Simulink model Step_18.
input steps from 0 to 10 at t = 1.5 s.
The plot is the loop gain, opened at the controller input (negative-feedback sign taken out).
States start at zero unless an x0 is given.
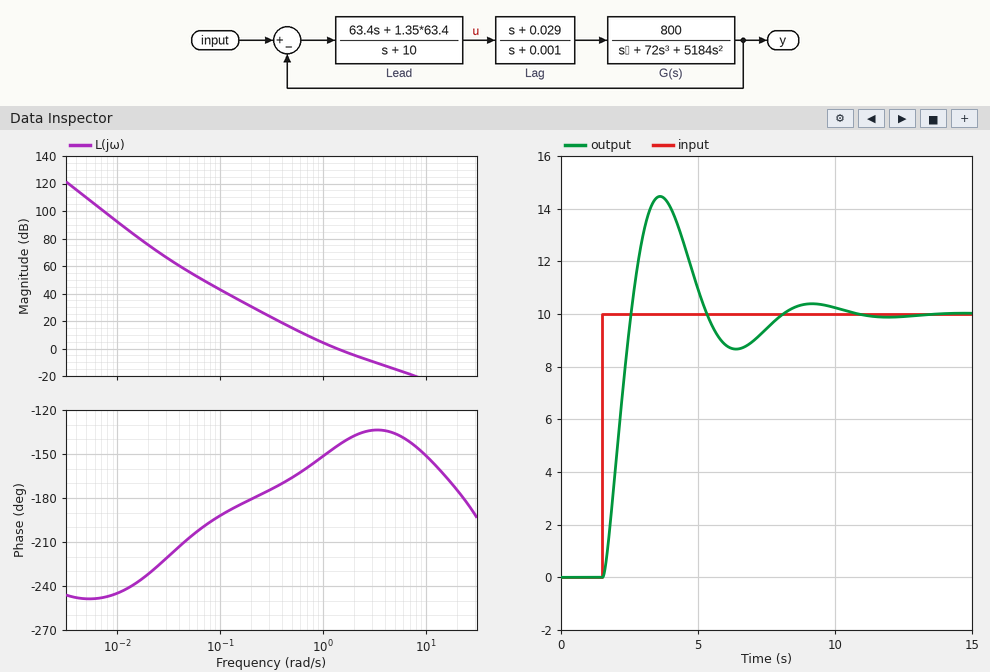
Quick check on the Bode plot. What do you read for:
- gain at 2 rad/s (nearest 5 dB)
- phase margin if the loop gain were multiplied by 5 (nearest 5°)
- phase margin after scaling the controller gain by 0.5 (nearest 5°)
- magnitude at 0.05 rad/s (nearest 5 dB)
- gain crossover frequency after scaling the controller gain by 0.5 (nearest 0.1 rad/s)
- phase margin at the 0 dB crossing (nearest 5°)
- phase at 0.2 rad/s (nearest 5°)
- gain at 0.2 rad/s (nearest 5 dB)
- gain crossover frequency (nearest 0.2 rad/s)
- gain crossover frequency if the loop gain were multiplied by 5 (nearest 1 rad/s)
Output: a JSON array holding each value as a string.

["-5 dB", "45°", "25°", "55 dB", "0.9 rad/s", "35°", "-180°", "30 dB", "1.4 rad/s", "5 rad/s"]
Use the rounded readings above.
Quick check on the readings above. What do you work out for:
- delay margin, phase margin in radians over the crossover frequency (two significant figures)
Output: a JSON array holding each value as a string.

["0.44 s"]
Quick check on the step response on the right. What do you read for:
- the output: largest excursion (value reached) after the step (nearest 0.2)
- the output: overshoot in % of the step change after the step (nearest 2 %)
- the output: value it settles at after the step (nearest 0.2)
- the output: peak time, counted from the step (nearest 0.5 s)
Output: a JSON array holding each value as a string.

["14.4", "44 %", "10.0", "2.0 s"]
